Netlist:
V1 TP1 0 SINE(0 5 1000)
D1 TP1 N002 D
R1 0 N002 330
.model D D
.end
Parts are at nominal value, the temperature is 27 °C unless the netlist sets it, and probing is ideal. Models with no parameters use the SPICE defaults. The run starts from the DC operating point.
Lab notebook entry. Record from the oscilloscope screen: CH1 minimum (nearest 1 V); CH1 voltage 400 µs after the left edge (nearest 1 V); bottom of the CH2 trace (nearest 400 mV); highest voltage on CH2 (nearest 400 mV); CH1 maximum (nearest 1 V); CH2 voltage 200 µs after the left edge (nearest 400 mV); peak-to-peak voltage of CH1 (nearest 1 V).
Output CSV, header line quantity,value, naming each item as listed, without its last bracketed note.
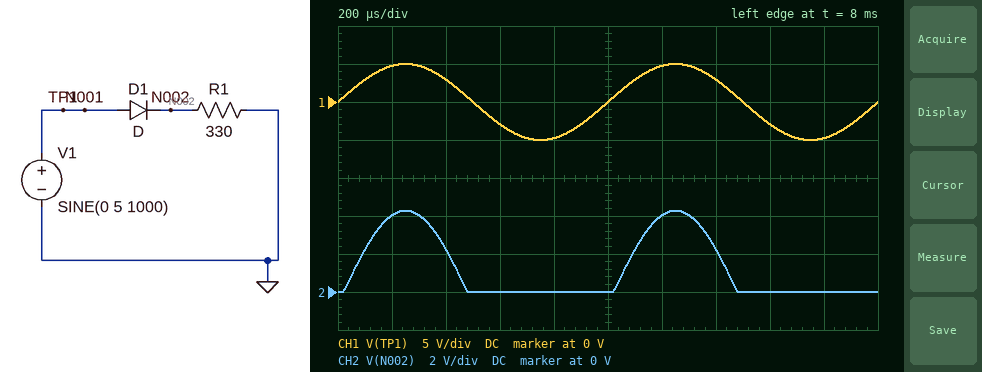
quantity,value
CH1 minimum,-5 V
CH1 voltage 400 µs after the left edge,3 V
bottom of the CH2 trace,0 V
highest voltage on CH2,4.4 V
CH1 maximum,5 V
CH2 voltage 200 µs after the left edge,4.0 V
peak-to-peak voltage of CH1,10 V
